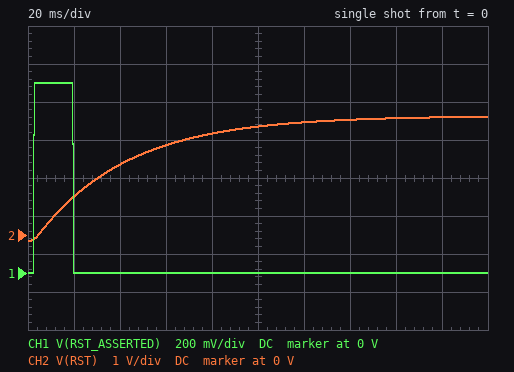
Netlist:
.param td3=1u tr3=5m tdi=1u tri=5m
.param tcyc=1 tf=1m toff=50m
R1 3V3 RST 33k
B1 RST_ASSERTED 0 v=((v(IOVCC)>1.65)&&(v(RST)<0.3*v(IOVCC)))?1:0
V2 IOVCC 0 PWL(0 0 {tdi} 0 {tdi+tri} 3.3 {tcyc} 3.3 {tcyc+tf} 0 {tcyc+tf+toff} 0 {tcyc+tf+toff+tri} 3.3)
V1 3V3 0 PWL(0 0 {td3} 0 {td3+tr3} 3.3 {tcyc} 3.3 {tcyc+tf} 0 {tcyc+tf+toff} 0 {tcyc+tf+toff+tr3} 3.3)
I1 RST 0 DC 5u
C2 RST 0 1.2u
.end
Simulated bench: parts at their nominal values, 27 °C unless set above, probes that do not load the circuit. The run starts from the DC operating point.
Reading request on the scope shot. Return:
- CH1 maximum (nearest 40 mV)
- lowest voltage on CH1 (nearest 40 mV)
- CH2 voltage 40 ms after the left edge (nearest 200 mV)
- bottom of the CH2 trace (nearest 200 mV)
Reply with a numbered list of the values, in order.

1. 1.00 V
2. 0 V
3. 1.8 V
4. -200 mV
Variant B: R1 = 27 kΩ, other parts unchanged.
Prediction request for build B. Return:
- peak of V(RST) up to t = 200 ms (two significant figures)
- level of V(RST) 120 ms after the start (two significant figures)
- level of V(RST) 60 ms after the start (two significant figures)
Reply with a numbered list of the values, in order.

1. 3.2 V
2. 3.1 V
3. 2.6 V
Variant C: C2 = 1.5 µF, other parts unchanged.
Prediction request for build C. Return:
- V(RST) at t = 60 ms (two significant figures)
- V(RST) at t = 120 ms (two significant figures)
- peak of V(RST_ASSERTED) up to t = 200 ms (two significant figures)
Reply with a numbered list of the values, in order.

1. 2.1 V
2. 2.8 V
3. 1.0 V
